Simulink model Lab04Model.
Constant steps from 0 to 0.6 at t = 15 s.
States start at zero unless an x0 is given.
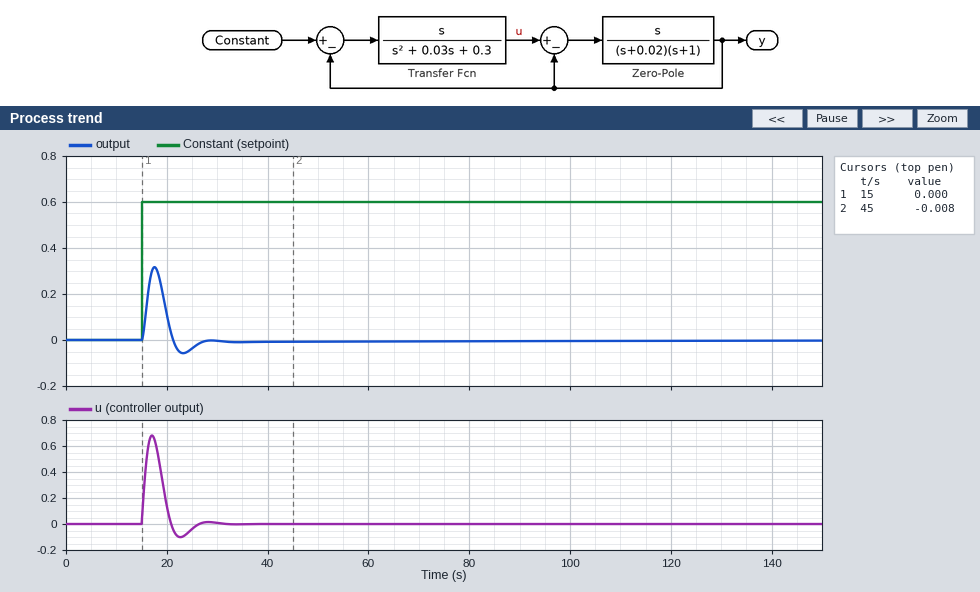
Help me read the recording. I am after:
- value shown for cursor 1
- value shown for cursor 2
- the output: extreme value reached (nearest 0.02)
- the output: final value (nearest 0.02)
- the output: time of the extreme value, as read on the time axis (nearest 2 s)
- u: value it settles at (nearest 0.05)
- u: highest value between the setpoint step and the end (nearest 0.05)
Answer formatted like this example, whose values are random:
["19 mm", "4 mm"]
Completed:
["0.000", "-0.008", "0.32", "0.00", "18 s", "0.00", "0.70"]
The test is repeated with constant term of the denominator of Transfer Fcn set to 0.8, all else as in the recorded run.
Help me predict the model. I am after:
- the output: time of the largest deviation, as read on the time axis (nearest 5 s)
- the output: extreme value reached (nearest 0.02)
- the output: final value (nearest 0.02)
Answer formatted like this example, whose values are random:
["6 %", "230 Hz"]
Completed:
["15 s", "0.22", "0.00"]
